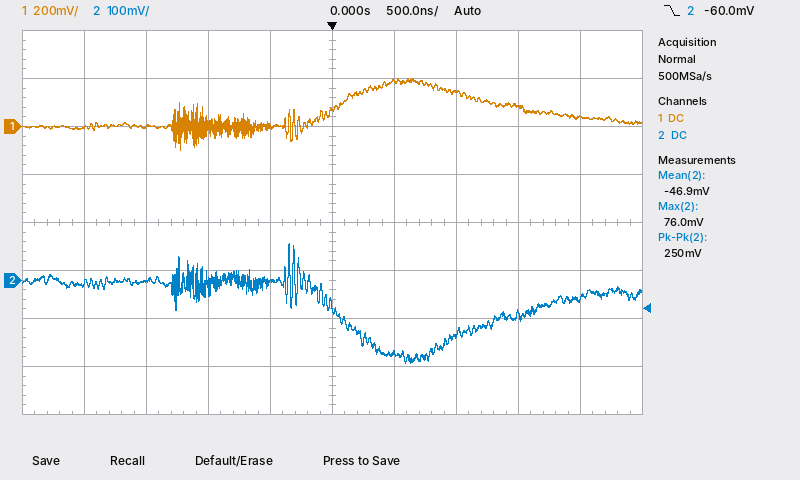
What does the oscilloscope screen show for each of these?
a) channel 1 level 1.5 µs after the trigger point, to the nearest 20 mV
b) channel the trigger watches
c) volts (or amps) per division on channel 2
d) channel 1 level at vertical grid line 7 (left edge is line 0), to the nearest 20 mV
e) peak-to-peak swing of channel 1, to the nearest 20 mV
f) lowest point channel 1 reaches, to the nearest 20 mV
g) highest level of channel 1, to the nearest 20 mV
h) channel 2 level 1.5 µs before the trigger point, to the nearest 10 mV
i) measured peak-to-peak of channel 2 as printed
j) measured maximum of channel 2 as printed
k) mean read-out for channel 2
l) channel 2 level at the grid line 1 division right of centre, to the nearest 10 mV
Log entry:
80 mV
channel 2
100 mV
140 mV
300 mV
-100 mV
200 mV
0 mV
250 mV
76.0 mV
-46.9 mV
-150 mV
